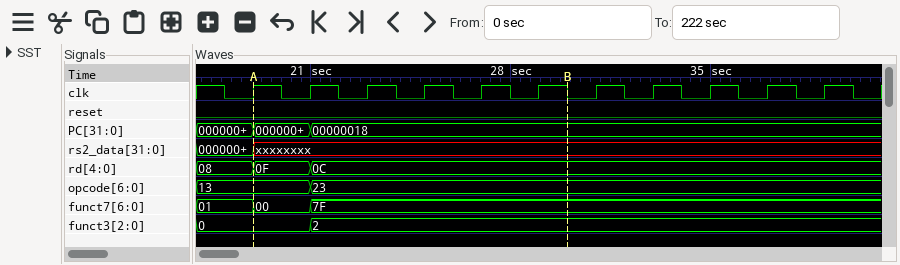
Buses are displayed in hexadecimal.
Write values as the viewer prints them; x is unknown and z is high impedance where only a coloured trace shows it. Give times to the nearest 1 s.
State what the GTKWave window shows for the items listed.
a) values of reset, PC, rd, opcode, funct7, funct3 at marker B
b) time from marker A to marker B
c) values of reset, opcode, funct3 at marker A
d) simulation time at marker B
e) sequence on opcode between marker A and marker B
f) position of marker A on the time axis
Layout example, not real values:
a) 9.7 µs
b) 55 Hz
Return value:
a) reset=0, PC=00000018, rd=0C, opcode=23, funct7=7F, funct3=2
b) 11 s
c) reset=0, opcode=13, funct3=0
d) 30 s
e) 13, 23
f) 19 s
